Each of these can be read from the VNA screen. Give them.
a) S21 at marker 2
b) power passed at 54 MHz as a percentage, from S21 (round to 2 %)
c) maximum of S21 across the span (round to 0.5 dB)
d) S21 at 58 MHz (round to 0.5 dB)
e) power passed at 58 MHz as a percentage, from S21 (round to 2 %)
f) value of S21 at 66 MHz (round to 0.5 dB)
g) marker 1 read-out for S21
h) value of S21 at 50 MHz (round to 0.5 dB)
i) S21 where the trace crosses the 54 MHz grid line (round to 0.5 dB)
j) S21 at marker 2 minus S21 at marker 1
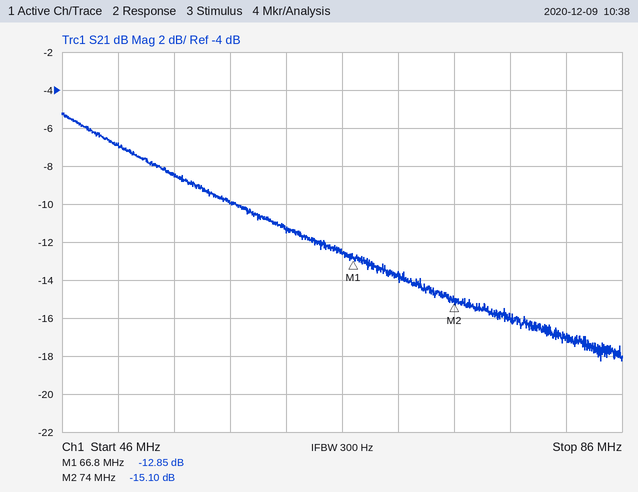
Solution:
-15.10 dB
14 %
-5.0 dB
-10.0 dB
10 %
-12.5 dB
-12.85 dB
-7.0 dB
-8.5 dB
-2.25 dB
